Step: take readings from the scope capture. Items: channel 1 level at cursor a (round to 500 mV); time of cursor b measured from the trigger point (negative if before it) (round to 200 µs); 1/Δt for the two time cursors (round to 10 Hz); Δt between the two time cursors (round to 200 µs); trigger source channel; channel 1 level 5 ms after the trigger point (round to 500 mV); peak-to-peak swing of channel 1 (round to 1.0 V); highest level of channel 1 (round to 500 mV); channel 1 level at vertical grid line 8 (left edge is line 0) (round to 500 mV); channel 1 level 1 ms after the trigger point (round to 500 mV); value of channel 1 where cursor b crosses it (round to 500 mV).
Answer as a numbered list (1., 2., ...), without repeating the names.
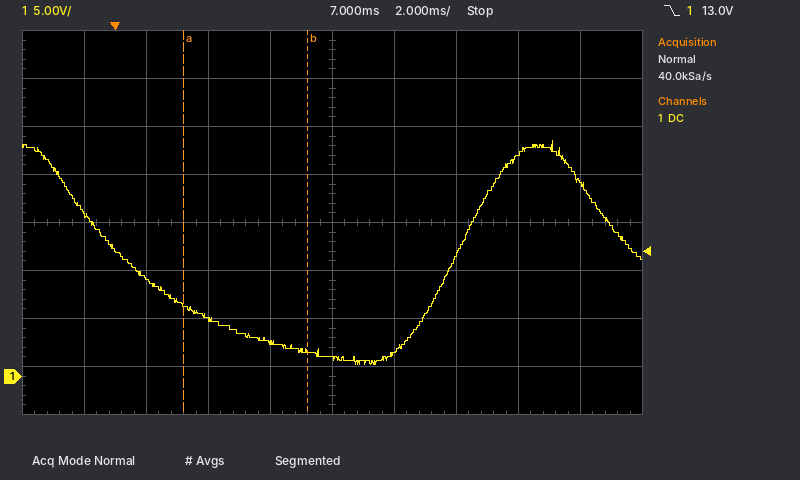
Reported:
1. 7.5 V
2. +6.2 ms
3. 250 Hz
4. 4.0 ms
5. channel 1
6. 3.5 V
7. 23.0 V
8. 24.5 V
9. 23.0 V
10. 10.0 V
11. 2.5 V
